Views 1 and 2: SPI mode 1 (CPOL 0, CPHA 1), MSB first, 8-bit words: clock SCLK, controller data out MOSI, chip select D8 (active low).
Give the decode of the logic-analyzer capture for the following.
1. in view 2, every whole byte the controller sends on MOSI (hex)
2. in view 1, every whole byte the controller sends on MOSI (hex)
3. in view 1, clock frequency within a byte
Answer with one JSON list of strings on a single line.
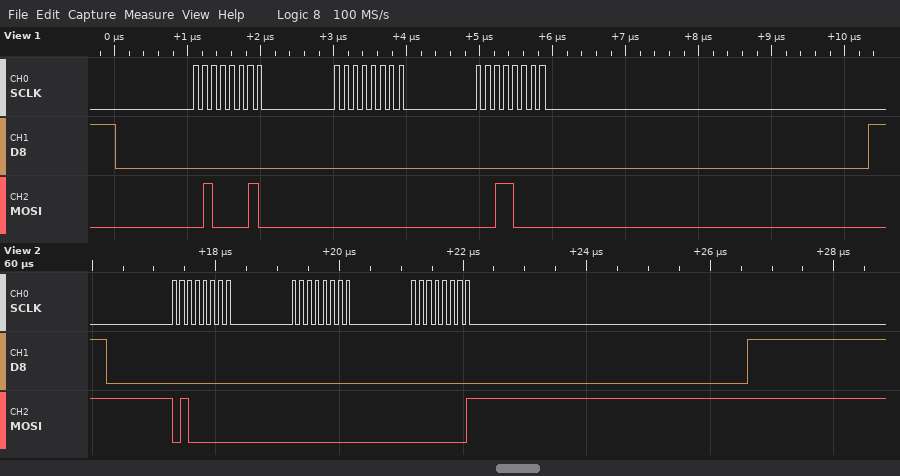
["40 00 01", "42 00 30", "8 MHz"]
